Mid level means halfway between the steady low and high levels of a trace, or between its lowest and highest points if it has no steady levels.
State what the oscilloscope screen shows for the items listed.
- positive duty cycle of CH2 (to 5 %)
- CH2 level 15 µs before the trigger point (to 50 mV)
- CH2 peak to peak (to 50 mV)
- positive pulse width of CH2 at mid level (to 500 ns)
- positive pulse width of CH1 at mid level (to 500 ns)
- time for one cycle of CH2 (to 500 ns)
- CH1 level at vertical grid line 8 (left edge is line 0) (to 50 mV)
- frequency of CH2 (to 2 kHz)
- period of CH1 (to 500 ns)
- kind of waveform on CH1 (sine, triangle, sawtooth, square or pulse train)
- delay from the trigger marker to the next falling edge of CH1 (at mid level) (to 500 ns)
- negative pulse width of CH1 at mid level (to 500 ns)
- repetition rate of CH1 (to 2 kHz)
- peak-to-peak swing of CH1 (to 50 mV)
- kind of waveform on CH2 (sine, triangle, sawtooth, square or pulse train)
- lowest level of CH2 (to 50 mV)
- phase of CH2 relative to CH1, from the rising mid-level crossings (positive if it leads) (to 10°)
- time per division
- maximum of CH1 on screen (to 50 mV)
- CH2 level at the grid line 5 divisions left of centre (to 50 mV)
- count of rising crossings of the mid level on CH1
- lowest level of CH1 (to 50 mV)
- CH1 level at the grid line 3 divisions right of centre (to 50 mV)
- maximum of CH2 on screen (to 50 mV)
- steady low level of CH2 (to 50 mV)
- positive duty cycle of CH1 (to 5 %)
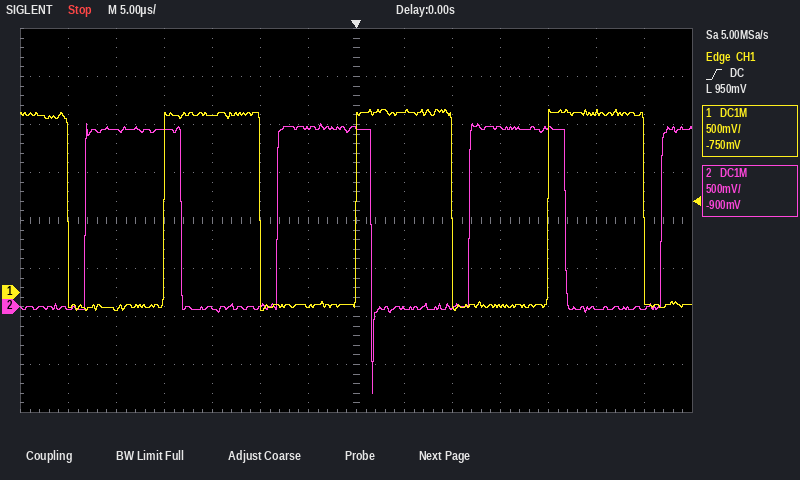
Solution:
50 %
0 mV
2.80 V
10.0 µs
10.0 µs
20.0 µs
1.90 V
50 kHz
20.0 µs
square
10.0 µs
10.0 µs
50 kHz
2.10 V
square
-900 mV
+150°
5 µs
1.90 V
1.85 V
3
-200 mV
-150 mV
1.90 V
0 mV
50 %
